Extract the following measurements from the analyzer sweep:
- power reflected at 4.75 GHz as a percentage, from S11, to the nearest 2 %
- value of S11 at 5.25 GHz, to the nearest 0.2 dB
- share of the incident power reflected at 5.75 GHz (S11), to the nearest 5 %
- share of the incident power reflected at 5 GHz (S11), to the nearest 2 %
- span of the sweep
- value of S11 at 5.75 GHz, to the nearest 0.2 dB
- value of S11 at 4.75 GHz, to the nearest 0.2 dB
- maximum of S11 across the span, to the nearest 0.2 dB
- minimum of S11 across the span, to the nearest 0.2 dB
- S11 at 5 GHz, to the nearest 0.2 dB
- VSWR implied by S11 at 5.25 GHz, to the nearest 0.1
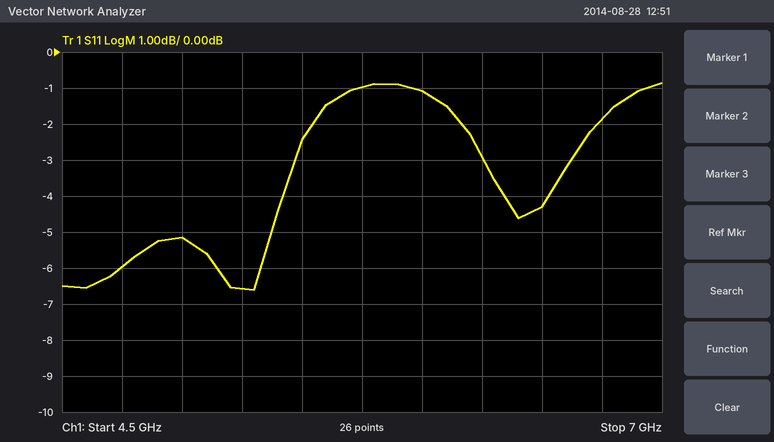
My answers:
26 %
-6.6 dB
80 %
30 %
2.5 GHz
-1.0 dB
-6.0 dB
-0.8 dB
-6.6 dB
-5.2 dB
2.8
